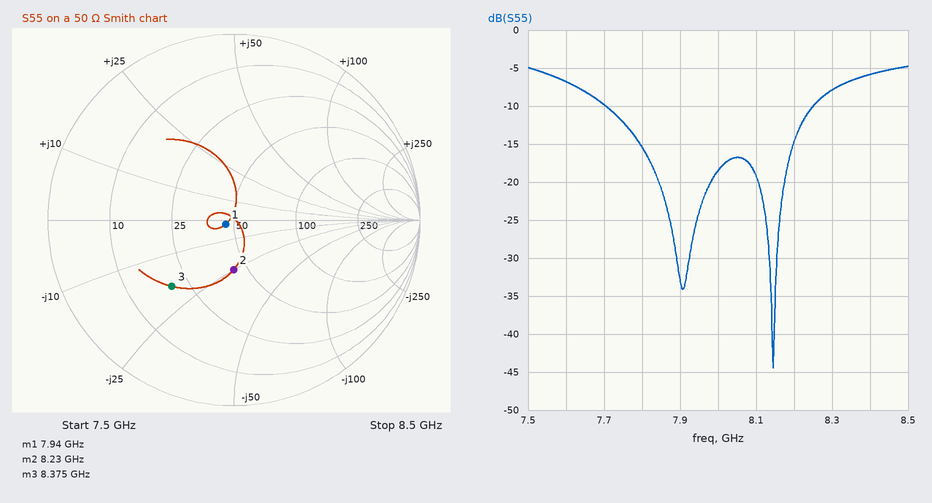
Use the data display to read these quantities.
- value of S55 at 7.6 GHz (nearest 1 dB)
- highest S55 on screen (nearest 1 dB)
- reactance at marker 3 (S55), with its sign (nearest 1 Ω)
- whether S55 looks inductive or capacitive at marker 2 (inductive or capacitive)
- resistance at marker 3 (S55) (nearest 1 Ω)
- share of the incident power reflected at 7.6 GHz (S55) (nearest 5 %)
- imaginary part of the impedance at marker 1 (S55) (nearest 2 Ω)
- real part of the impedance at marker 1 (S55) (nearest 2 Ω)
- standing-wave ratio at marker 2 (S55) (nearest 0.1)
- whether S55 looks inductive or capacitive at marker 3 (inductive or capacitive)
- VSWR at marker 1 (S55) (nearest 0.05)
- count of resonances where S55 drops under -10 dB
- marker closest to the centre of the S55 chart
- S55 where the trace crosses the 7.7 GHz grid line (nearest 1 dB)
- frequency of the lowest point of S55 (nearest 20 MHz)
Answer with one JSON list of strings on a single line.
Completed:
["-7 dB", "-5 dB", "-19 Ω", "capacitive", "20 Ω", "20 %", "-2 Ω", "46 Ω", "1.7", "capacitive", "1.10", "2", "marker 1", "-10 dB", "8.14 GHz"]
